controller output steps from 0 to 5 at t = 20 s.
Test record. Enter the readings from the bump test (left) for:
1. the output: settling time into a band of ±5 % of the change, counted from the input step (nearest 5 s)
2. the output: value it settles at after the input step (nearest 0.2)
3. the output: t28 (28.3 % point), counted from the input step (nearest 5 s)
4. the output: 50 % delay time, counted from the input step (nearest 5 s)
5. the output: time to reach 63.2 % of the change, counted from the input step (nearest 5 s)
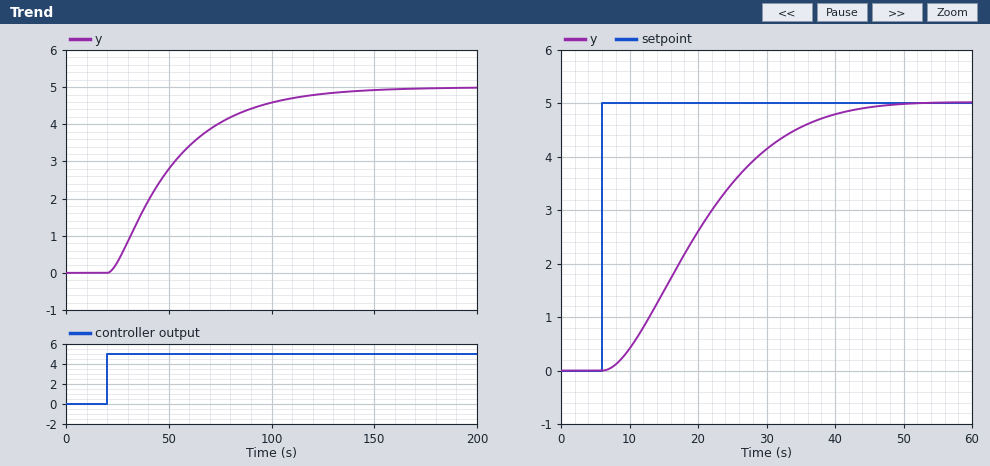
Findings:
95 s
5.0
15 s
25 s
35 s
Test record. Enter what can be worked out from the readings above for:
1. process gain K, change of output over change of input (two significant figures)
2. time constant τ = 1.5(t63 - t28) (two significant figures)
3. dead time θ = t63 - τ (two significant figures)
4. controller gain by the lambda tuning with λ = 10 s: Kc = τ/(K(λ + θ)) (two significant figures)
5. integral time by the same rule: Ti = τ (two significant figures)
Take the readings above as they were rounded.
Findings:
1.0
30 s
5.0 s
2.0
30 s
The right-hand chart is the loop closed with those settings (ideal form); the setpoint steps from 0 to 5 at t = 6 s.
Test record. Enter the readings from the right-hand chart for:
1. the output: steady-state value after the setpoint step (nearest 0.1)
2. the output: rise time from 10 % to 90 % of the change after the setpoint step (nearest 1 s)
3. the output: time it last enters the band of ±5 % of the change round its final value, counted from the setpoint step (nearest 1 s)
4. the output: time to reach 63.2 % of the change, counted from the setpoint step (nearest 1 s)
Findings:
5.0
24 s
33 s
17 s
